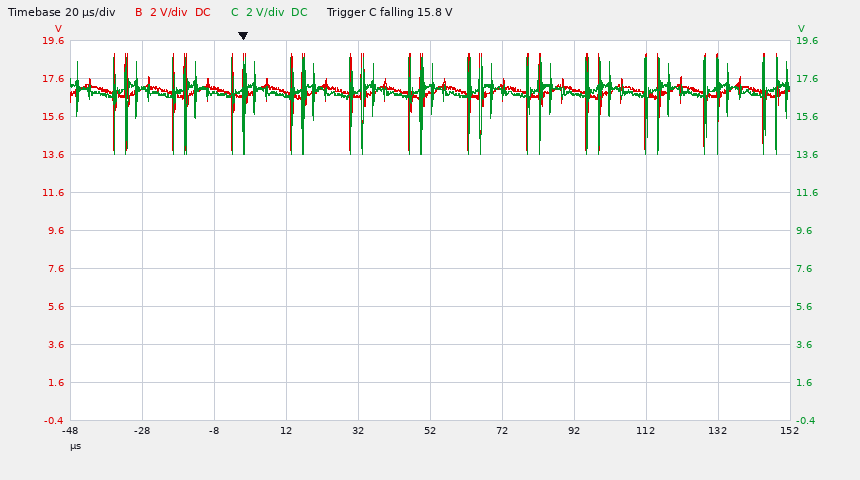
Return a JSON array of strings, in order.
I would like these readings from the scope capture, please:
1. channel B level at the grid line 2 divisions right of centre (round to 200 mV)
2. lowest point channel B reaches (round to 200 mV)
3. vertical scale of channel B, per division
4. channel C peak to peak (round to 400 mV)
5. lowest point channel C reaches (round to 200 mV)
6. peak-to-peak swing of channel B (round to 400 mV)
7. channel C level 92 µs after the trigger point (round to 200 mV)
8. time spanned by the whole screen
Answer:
["17.0 V", "13.8 V", "2 V", "5.2 V", "13.6 V", "5.2 V", "16.8 V", "200 µs"]
